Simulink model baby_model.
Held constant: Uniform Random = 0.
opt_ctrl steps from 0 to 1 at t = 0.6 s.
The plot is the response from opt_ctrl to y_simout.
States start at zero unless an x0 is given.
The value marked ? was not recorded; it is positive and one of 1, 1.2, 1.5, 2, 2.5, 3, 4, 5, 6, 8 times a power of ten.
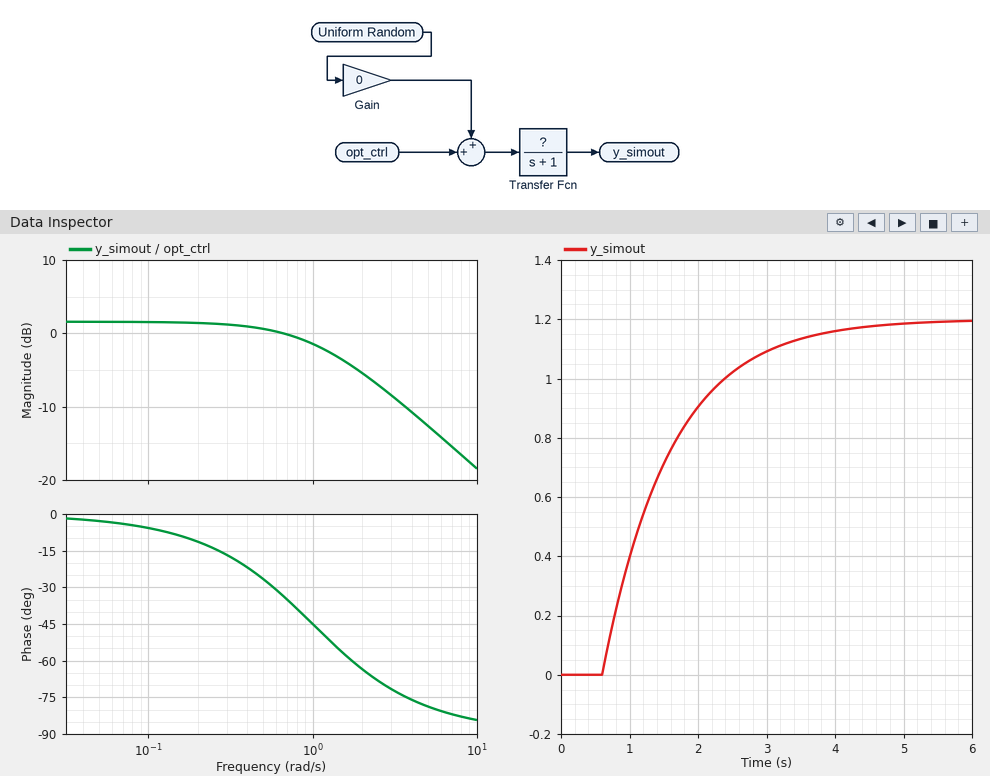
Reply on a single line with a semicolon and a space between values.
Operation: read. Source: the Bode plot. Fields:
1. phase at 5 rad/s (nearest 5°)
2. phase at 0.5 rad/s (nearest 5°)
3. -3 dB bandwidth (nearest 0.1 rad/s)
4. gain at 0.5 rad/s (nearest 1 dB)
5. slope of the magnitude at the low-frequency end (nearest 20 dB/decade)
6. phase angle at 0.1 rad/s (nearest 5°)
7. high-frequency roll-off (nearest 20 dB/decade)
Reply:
-80°; -25°; 1.0 rad/s; 1 dB; 0 dB/decade; -5°; -20 dB/decade
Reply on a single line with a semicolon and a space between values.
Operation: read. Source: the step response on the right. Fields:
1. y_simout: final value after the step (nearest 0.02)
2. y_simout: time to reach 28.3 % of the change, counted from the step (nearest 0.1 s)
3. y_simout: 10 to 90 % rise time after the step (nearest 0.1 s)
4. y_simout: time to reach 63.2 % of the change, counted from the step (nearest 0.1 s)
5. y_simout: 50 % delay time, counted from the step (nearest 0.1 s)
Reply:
1.20; 0.3 s; 2.2 s; 1.0 s; 0.7 s
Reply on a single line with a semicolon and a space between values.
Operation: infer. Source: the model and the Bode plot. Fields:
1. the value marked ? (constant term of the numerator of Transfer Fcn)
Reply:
1.2
